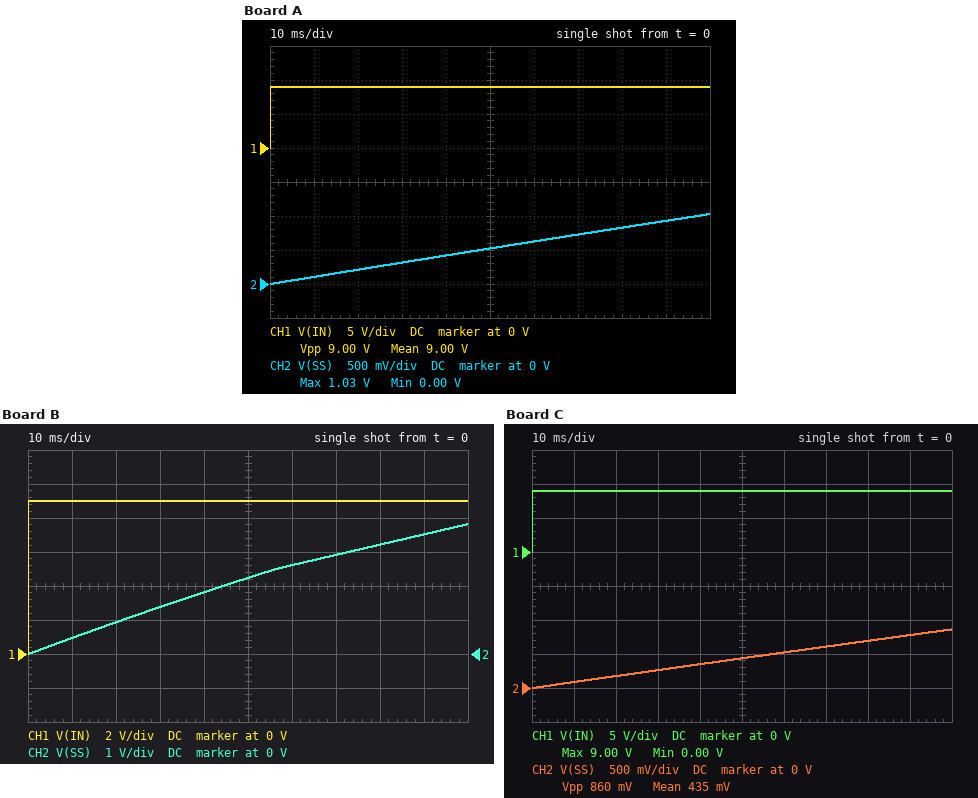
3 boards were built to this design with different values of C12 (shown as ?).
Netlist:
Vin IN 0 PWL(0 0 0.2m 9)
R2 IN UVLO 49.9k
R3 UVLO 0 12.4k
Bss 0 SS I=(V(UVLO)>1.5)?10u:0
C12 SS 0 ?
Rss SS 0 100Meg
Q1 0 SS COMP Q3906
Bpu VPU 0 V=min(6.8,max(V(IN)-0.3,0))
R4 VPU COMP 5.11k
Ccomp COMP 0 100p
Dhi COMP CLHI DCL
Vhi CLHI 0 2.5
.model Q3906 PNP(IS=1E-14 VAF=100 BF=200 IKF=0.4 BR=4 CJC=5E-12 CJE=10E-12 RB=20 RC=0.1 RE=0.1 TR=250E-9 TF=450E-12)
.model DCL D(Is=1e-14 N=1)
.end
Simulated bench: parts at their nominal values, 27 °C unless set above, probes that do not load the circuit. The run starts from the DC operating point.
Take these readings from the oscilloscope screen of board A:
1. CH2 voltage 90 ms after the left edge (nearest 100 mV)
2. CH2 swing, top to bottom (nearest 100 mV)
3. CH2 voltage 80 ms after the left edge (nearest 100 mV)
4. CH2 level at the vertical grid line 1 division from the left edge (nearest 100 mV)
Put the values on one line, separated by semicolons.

900 mV; 1.0 V; 800 mV; 100 mV
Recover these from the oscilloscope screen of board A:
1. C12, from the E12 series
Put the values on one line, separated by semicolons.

1.5 µF
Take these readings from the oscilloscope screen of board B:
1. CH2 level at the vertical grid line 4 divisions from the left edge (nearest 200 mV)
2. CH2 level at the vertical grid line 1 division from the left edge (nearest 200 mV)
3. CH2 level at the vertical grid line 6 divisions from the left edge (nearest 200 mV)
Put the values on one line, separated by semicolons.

1.8 V; 400 mV; 2.6 V
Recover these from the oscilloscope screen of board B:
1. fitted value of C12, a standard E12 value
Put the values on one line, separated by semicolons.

330 nF
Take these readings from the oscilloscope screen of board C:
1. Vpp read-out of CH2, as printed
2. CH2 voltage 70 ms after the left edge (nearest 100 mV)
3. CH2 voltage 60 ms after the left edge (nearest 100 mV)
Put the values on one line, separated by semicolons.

860 mV; 600 mV; 500 mV
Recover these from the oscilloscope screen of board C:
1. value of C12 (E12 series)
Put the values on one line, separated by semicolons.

1.8 µF
